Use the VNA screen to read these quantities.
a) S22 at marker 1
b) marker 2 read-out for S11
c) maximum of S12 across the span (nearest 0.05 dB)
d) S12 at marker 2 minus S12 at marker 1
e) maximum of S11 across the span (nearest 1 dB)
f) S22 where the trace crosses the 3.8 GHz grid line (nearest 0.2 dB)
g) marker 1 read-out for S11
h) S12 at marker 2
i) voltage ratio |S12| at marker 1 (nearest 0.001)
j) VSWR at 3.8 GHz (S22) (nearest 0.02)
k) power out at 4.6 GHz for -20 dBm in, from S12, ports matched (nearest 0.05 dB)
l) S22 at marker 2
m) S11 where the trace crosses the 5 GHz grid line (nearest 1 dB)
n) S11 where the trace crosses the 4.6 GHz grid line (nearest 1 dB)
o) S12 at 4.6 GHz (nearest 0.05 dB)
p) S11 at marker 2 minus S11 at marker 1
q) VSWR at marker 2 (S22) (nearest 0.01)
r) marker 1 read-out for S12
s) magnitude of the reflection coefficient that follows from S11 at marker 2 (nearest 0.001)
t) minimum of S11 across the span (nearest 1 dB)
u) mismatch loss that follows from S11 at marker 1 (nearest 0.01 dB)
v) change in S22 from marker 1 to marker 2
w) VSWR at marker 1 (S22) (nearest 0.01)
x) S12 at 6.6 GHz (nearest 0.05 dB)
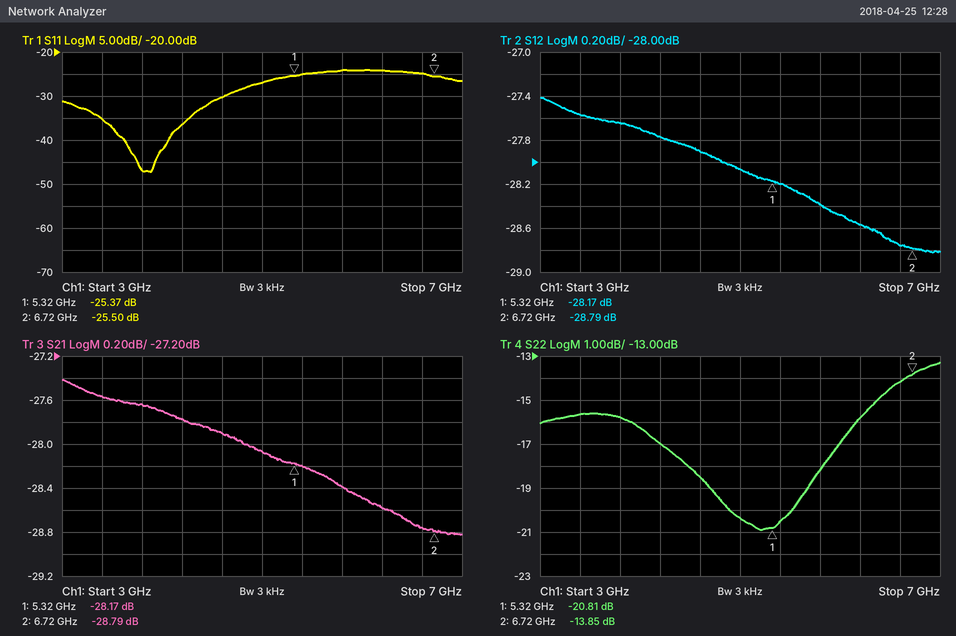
-20.81 dB
-25.50 dB
-27.40 dB
-0.62 dB
-24 dB
-15.8 dB
-25.37 dB
-28.79 dB
0.039
1.38
-47.90 dBm
-13.85 dB
-27 dB
-30 dB
-27.90 dB
-0.13 dB
1.51
-28.17 dB
0.053
-47 dB
0.01 dB
6.96 dB
1.20
-28.75 dB
